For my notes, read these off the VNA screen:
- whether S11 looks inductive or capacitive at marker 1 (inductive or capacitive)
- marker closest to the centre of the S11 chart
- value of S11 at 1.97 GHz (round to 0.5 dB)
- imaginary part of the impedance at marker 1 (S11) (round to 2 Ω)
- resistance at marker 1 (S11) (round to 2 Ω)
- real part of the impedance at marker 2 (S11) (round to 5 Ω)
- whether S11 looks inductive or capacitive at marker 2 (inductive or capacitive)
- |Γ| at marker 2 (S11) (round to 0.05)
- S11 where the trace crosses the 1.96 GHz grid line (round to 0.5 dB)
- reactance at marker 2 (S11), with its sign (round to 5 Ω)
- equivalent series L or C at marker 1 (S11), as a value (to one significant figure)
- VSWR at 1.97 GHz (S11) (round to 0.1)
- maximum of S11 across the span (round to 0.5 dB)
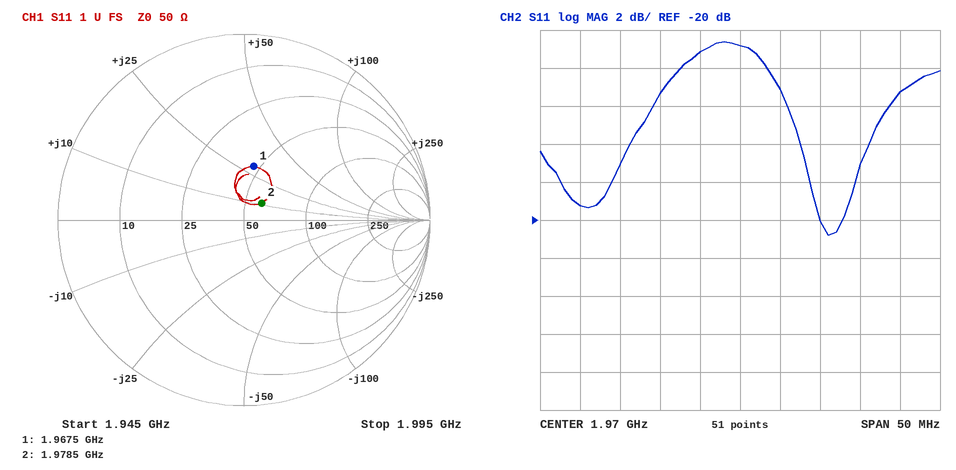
inductive
marker 2
-11.0 dB
+30 Ω
46 Ω
60 Ω
inductive
0.15
-13.5 dB
+10 Ω
2 nH
1.8
-10.5 dB
